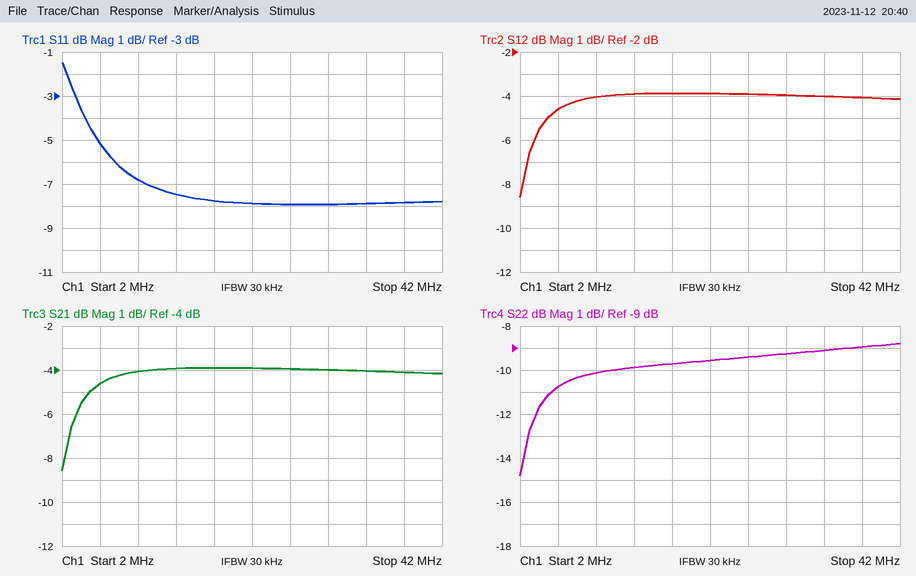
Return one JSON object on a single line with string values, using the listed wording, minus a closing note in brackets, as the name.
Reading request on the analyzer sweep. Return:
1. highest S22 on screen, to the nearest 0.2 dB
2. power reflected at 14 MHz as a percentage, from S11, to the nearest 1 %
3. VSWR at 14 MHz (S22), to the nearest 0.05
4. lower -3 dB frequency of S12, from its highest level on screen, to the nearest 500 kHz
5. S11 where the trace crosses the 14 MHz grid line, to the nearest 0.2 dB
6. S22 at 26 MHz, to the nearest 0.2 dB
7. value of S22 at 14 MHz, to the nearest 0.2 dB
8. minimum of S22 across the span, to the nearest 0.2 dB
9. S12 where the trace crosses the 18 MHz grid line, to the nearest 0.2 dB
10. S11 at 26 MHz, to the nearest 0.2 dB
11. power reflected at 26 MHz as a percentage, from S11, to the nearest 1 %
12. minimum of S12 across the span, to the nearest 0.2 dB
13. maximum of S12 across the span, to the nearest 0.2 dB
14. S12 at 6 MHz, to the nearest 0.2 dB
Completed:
{"highest S22 on screen, to the nearest 0.2 dB": "-8.8 dB", "power reflected at 14 MHz as a percentage, from S11, to the nearest 1 %": "18 %", "VSWR at 14 MHz (S22), to the nearest 0.05": "1.95", "lower -3 dB frequency of S12, from its highest level on screen, to the nearest 500 kHz": "3.0 MHz", "S11 where the trace crosses the 14 MHz grid line, to the nearest 0.2 dB": "-7.4 dB", "S22 at 26 MHz, to the nearest 0.2 dB": "-9.4 dB", "value of S22 at 14 MHz, to the nearest 0.2 dB": "-9.8 dB", "minimum of S22 across the span, to the nearest 0.2 dB": "-14.8 dB", "S12 where the trace crosses the 18 MHz grid line, to the nearest 0.2 dB": "-3.8 dB", "S11 at 26 MHz, to the nearest 0.2 dB": "-8.0 dB", "power reflected at 26 MHz as a percentage, from S11, to the nearest 1 %": "16 %", "minimum of S12 across the span, to the nearest 0.2 dB": "-8.6 dB", "maximum of S12 across the span, to the nearest 0.2 dB": "-3.8 dB", "S12 at 6 MHz, to the nearest 0.2 dB": "-4.6 dB"}
